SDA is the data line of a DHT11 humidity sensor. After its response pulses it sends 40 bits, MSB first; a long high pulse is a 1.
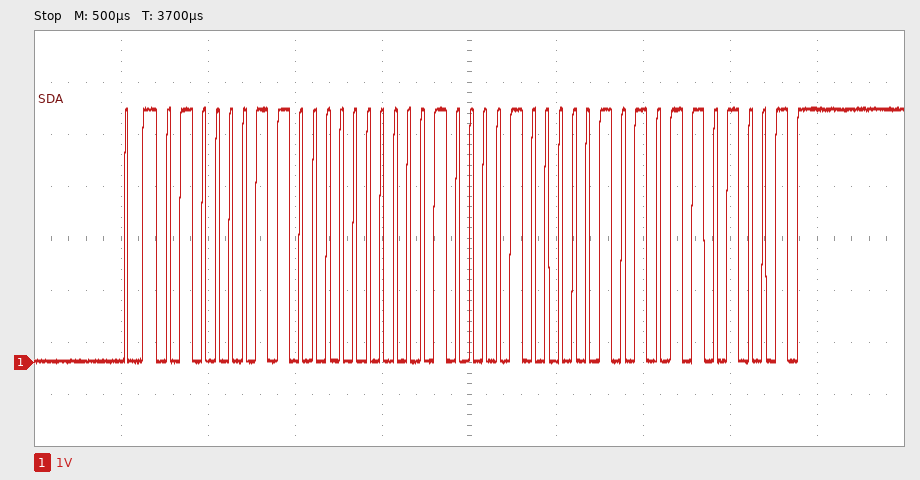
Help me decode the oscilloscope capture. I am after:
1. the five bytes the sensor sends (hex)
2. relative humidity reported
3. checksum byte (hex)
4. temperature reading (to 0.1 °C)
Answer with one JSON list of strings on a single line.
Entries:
["43 00 21 05 69", "67 %", "0x69", "33.5 °C"]
